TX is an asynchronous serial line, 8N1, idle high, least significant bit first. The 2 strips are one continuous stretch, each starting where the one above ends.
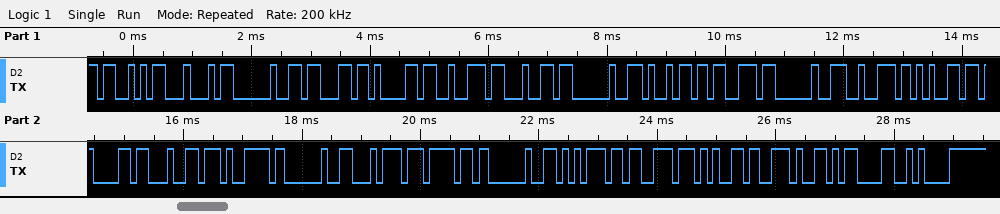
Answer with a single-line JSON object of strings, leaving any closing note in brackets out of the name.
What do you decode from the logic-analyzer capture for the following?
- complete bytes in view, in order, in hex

{"complete bytes in view, in order, in hex": "53 44 20 63 61 72 64 20 69 73 20 72 65 61 64 79 20 74 6F 20 75 73 65 2E 0D 0A"}
